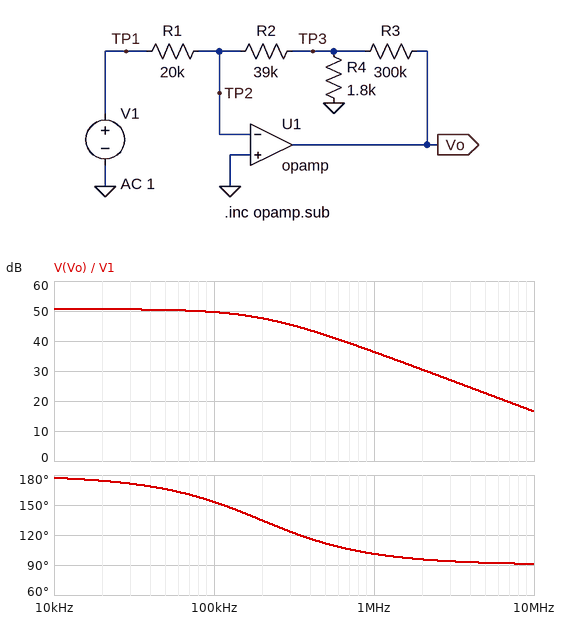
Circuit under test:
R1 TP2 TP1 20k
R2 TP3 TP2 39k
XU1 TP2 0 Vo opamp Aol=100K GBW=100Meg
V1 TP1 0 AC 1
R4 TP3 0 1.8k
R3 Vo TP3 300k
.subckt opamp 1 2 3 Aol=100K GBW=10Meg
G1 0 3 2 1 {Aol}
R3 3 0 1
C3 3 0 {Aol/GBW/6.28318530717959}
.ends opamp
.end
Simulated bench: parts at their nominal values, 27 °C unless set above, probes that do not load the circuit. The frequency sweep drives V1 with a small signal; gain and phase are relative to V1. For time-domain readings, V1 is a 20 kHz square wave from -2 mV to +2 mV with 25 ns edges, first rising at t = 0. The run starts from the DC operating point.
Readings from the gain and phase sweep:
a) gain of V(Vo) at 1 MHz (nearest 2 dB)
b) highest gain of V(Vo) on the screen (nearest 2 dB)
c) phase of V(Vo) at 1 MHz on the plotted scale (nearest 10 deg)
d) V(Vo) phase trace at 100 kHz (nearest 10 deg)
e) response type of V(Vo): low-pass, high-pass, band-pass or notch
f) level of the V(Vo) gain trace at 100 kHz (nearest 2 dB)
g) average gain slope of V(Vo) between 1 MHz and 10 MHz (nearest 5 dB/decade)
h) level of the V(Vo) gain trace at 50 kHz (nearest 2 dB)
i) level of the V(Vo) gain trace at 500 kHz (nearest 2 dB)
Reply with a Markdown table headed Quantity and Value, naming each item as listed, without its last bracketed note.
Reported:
| Quantity | Value |
|---|---|
| gain of V(Vo) at 1 MHz | 36 dB |
| highest gain of V(Vo) on the screen | 50 dB |
| phase of V(Vo) at 1 MHz on the plotted scale | 100 deg |
| V(Vo) phase trace at 100 kHz | 150 deg |
| response type of V(Vo): low-pass, high-pass, band-pass or notch | low-pass |
| level of the V(Vo) gain trace at 100 kHz | 50 dB |
| average gain slope of V(Vo) between 1 MHz and 10 MHz | -20 dB/decade |
| level of the V(Vo) gain trace at 50 kHz | 50 dB |
| level of the V(Vo) gain trace at 500 kHz | 42 dB |
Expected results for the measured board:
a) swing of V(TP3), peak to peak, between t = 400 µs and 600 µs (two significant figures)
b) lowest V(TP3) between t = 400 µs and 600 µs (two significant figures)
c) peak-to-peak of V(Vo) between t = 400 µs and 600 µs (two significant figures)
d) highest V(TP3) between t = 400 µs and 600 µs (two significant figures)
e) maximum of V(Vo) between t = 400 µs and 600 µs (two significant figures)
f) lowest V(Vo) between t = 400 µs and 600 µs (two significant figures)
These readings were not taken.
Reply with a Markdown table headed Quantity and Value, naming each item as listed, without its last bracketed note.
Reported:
| Quantity | Value |
|---|---|
| swing of V(TP3), peak to peak, between t = 400 µs and 600 µs | 7.8 mV |
| lowest V(TP3) between t = 400 µs and 600 µs | -3.9 mV |
| peak-to-peak of V(Vo) between t = 400 µs and 600 µs | 1.4 V |
| highest V(TP3) between t = 400 µs and 600 µs | 3.9 mV |
| maximum of V(Vo) between t = 400 µs and 600 µs | 680 mV |
| lowest V(Vo) between t = 400 µs and 600 µs | -680 mV |
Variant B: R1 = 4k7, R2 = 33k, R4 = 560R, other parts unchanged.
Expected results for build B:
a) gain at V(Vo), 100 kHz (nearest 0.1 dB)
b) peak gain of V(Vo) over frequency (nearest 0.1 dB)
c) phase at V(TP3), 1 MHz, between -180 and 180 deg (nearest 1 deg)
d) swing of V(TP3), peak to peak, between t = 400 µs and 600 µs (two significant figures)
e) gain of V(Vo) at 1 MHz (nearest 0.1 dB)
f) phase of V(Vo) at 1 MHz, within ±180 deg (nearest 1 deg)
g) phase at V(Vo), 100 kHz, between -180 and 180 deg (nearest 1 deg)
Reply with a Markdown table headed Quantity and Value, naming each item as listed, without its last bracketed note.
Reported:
| Quantity | Value |
|---|---|
| gain at V(Vo), 100 kHz | 58.6 dB |
| peak gain of V(Vo) over frequency | 71.3 dB |
| phase at V(TP3), 1 MHz, between -180 and 180 deg | 86 deg |
| swing of V(TP3), peak to peak, between t = 400 µs and 600 µs | 26 mV |
| gain of V(Vo) at 1 MHz | 38.9 dB |
| phase of V(Vo) at 1 MHz, within ±180 deg | 91 deg |
| phase at V(Vo), 100 kHz, between -180 and 180 deg | 103 deg |
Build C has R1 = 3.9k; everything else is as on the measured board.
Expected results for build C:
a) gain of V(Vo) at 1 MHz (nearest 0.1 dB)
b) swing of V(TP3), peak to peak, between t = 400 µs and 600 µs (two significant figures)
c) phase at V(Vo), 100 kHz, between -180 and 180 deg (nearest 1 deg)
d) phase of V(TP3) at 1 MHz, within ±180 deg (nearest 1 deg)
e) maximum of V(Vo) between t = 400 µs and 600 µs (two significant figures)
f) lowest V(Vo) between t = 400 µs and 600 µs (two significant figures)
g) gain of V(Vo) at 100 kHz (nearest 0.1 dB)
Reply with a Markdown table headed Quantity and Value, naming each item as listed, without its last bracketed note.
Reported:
| Quantity | Value |
|---|---|
| gain of V(Vo) at 1 MHz | 39.2 dB |
| swing of V(TP3), peak to peak, between t = 400 µs and 600 µs | 39 mV |
| phase at V(Vo), 100 kHz, between -180 and 180 deg | 118 deg |
| phase of V(TP3) at 1 MHz, within ±180 deg | 89 deg |
| maximum of V(Vo) between t = 400 µs and 600 µs | 3.4 V |
| lowest V(Vo) between t = 400 µs and 600 µs | -3.4 V |
| gain of V(Vo) at 100 kHz | 58.1 dB |
